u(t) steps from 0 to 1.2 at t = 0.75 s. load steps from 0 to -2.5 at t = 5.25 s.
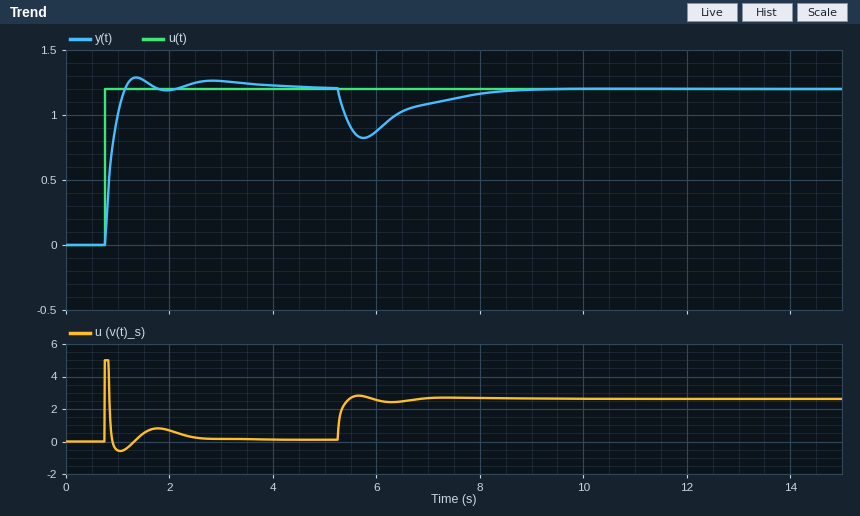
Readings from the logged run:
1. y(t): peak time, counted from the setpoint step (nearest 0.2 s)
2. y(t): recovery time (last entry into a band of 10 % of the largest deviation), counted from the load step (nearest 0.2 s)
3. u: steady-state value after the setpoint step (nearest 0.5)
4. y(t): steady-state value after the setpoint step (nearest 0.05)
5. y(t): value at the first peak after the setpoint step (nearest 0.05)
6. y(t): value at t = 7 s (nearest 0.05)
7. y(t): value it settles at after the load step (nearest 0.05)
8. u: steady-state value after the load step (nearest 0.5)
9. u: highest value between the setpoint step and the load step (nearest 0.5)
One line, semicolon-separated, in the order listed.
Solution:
0.6 s; 2.8 s; 0.0; 1.20; 1.30; 1.10; 1.20; 2.5; 5.0
